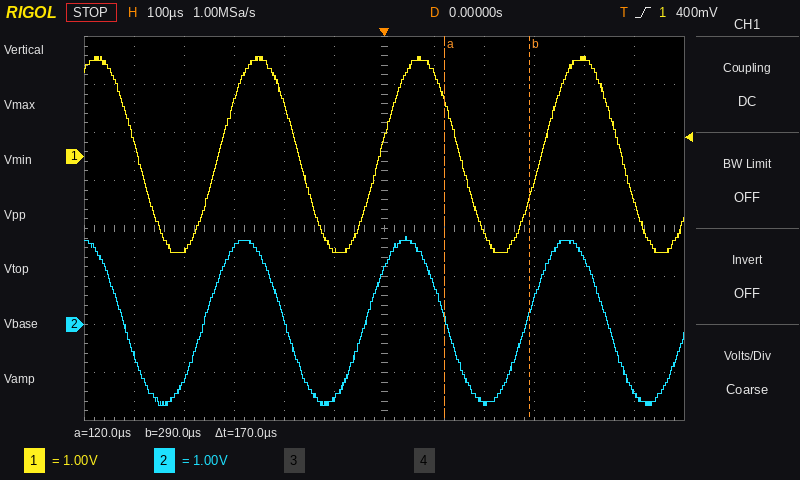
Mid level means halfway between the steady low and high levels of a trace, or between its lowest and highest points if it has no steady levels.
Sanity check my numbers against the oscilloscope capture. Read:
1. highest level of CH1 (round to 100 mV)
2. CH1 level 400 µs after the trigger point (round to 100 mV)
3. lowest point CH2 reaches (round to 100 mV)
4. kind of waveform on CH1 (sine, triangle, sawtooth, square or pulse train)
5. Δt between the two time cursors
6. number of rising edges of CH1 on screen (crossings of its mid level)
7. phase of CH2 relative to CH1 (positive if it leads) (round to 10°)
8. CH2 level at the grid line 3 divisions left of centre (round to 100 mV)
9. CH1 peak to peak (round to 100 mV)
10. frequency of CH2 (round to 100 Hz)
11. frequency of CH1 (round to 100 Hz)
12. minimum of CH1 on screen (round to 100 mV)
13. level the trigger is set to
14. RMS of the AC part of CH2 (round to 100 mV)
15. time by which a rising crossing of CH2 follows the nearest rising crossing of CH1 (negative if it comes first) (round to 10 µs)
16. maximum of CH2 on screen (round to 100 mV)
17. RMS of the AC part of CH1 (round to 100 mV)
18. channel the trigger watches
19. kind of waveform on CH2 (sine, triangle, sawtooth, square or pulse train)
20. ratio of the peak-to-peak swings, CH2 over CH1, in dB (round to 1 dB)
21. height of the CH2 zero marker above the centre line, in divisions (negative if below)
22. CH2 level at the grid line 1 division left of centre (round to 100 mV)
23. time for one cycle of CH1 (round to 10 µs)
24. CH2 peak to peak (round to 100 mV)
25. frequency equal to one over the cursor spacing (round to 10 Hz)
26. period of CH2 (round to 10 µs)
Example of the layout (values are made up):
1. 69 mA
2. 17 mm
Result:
1. 2.1 V
2. 2.0 V
3. -1.7 V
4. sine
5. 170 µs
6. 3
7. +30°
8. 1.6 V
9. 4.1 V
10. 3.1 kHz
11. 3.1 kHz
12. -2.0 V
13. 400 mV
14. 1.2 V
15. -30 µs
16. 1.8 V
17. 1.4 V
18. CH1
19. sine
20. -1 dB
21. -2.0 div
22. -1.5 V
23. 320 µs
24. 3.5 V
25. 5.88 kHz
26. 320 µs
